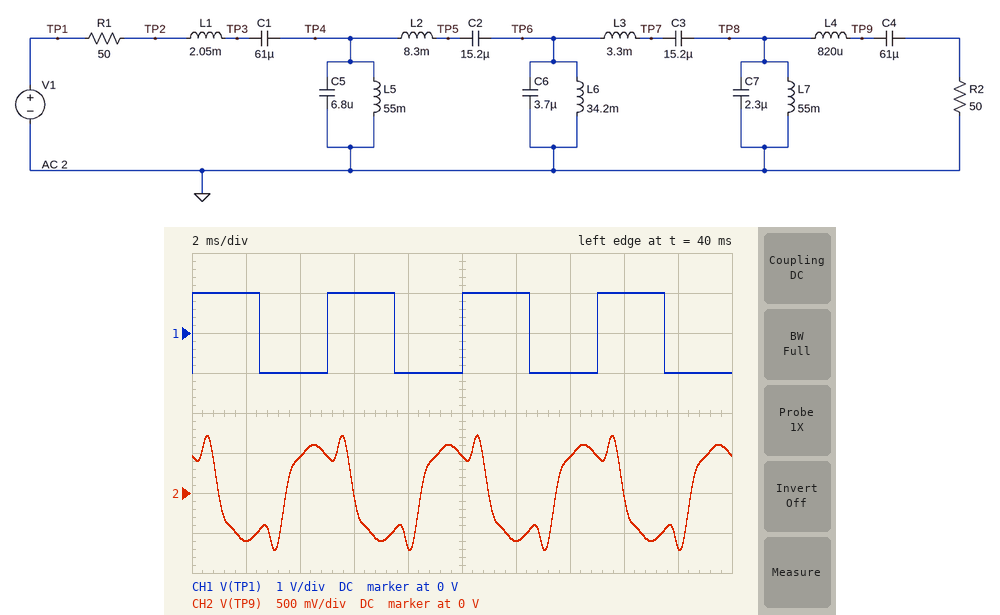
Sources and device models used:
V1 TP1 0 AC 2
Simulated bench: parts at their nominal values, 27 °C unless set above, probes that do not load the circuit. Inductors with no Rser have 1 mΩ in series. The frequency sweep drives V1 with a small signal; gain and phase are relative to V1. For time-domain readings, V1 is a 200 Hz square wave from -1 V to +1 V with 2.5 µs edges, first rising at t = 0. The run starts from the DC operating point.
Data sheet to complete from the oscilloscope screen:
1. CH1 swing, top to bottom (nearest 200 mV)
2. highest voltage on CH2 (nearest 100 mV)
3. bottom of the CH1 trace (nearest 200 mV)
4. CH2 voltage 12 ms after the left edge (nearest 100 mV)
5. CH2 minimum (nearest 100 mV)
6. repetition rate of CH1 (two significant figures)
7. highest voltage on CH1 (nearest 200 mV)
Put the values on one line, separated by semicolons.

2.0 V; 700 mV; -1.0 V; -600 mV; -700 mV; 200 Hz; 1.0 V
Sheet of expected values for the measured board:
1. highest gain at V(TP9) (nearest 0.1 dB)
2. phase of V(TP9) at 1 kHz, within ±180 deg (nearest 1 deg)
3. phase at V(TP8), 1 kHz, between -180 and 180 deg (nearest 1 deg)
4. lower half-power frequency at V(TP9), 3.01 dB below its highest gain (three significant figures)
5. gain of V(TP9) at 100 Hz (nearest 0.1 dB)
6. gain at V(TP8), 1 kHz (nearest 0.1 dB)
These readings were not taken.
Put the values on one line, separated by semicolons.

-5.7 dB; -137 deg; -131 deg; 109 Hz; -12.0 dB; -6.3 dB
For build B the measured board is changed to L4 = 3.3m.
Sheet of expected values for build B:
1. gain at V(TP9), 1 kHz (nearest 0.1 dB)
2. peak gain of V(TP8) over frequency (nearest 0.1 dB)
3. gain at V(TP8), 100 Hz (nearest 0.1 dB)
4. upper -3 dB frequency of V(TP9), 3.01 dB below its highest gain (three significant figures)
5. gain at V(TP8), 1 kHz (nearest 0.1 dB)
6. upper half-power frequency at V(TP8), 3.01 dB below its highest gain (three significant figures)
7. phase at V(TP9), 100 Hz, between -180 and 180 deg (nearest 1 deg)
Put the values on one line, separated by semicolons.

-6.7 dB; -5.8 dB; -12.3 dB; 1.29 kHz; -6.2 dB; 1.34 kHz; -38 deg
